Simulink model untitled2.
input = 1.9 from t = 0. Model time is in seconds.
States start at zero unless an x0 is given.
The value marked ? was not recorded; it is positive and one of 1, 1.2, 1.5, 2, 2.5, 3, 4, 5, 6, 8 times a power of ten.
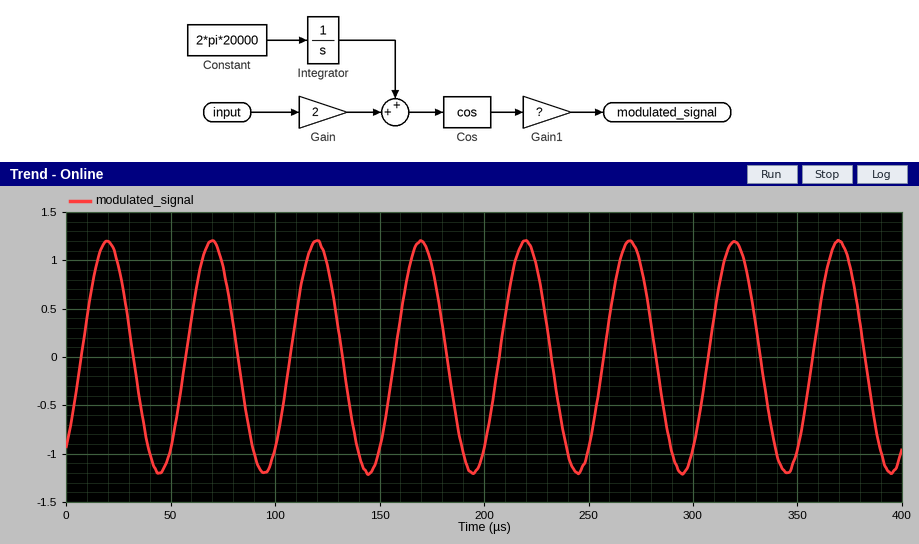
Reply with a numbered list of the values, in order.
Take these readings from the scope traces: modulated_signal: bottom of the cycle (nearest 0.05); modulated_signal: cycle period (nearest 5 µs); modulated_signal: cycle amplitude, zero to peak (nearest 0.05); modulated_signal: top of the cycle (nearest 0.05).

1. -1.20
2. 50 µs
3. 1.20
4. 1.20
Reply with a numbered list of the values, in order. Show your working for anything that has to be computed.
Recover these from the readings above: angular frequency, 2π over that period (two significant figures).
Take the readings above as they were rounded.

1. 2π / 50 = 0.13 rad/µs
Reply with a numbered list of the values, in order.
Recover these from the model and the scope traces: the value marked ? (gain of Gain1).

1. 1.2
